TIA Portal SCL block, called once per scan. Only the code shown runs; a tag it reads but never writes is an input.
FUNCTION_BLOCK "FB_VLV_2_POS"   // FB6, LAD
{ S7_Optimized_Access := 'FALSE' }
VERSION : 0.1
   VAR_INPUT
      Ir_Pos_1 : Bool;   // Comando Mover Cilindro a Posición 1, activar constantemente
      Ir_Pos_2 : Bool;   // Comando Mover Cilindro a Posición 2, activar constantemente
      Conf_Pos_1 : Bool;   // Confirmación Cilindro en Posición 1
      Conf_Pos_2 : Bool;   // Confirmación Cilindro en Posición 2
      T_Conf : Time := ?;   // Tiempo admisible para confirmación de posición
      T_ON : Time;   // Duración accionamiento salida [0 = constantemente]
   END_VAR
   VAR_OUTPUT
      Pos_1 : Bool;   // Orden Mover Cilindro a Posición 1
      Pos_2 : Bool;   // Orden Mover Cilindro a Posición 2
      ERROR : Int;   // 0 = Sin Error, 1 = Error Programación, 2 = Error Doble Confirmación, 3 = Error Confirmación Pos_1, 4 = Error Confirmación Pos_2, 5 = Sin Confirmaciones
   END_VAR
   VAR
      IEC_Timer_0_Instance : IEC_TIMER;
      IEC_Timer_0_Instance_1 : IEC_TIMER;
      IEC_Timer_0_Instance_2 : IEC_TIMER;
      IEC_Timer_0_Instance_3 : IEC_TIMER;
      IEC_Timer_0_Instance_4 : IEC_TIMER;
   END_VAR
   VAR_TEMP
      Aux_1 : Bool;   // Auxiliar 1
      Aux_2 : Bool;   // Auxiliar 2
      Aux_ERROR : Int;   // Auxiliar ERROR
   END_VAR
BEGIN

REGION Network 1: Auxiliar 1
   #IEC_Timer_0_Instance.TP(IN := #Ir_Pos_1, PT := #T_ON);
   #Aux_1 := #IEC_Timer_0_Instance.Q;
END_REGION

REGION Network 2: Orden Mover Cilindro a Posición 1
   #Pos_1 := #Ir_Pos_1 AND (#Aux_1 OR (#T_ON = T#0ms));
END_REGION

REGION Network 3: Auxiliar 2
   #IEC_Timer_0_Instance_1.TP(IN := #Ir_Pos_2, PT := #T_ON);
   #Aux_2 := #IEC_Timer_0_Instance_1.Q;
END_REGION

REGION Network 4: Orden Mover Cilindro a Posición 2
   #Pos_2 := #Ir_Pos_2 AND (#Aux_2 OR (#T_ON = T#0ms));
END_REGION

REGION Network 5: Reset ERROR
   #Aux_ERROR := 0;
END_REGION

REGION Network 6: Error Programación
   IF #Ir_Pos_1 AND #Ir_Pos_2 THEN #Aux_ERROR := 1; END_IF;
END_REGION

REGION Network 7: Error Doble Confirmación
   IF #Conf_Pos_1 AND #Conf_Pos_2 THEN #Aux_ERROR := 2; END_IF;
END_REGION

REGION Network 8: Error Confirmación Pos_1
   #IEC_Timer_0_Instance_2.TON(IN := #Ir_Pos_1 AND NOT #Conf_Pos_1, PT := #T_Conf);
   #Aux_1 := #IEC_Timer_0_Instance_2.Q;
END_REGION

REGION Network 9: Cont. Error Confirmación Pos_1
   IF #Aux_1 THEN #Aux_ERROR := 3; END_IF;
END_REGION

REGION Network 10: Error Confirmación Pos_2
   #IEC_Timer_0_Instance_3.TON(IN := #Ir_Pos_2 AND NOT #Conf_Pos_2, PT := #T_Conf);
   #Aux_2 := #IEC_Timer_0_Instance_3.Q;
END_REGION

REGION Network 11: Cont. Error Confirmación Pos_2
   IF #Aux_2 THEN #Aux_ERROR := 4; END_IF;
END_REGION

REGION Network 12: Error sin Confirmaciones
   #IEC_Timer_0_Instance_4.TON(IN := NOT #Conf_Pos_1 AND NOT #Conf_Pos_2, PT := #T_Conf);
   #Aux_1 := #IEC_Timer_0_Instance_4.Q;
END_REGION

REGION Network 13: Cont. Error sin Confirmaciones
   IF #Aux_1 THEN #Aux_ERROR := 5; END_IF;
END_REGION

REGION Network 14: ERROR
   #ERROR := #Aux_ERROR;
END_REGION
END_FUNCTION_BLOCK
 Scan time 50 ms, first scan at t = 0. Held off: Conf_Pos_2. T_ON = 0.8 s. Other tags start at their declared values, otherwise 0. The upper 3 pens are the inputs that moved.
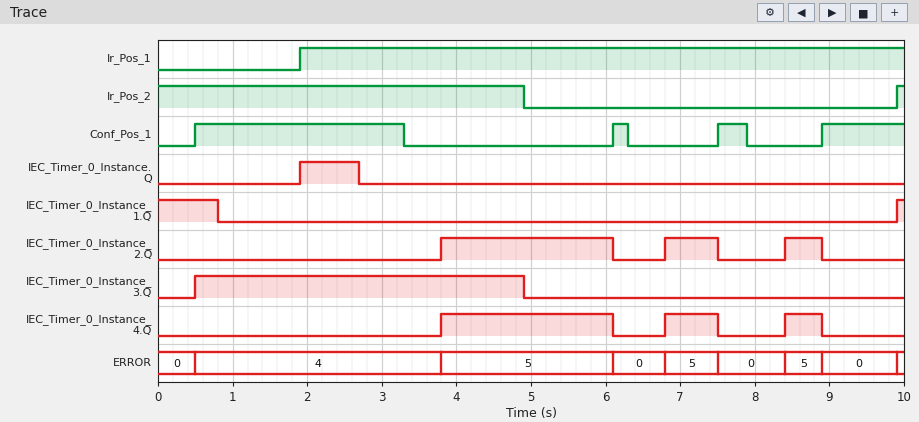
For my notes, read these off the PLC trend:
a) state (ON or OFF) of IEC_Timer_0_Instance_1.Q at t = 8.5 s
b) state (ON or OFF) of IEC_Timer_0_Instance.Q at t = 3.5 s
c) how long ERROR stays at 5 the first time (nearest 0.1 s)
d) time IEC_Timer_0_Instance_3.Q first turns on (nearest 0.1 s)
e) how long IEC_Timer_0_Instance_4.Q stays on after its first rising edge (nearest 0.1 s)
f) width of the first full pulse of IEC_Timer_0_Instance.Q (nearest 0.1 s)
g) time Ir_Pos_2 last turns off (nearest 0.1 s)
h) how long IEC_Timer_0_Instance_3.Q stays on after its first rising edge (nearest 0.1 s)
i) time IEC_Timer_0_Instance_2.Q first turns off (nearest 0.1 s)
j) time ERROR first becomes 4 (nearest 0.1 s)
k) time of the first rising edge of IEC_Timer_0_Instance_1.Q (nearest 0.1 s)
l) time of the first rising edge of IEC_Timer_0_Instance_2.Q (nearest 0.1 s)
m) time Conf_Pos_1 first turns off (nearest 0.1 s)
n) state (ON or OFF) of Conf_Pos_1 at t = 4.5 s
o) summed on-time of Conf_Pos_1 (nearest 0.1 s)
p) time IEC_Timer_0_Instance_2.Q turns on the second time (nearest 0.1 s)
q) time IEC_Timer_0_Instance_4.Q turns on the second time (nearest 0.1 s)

OFF
OFF
2.3 s
0.5 s
2.3 s
0.8 s
4.9 s
4.4 s
6.1 s
0.5 s
9.9 s
3.8 s
3.3 s
OFF
4.5 s
6.8 s
6.8 s
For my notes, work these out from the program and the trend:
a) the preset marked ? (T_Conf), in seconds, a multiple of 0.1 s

0.5 s
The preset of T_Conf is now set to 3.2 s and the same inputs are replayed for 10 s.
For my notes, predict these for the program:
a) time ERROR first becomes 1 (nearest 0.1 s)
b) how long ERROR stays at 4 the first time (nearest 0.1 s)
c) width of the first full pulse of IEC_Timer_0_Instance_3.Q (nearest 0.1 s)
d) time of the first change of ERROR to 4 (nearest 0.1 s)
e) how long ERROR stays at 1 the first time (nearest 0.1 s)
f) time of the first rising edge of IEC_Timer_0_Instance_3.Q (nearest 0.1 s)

1.9 s
1.7 s
1.7 s
3.2 s
1.3 s
3.2 s
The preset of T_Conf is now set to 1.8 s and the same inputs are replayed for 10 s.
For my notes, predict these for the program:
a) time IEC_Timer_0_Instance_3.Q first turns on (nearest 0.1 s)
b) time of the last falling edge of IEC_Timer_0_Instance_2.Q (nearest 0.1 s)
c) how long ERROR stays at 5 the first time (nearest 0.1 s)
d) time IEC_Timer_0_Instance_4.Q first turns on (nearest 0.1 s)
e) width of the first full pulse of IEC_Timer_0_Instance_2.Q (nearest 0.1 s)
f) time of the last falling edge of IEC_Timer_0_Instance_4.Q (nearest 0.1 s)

1.8 s
6.1 s
1.0 s
5.1 s
1.0 s
6.1 s
